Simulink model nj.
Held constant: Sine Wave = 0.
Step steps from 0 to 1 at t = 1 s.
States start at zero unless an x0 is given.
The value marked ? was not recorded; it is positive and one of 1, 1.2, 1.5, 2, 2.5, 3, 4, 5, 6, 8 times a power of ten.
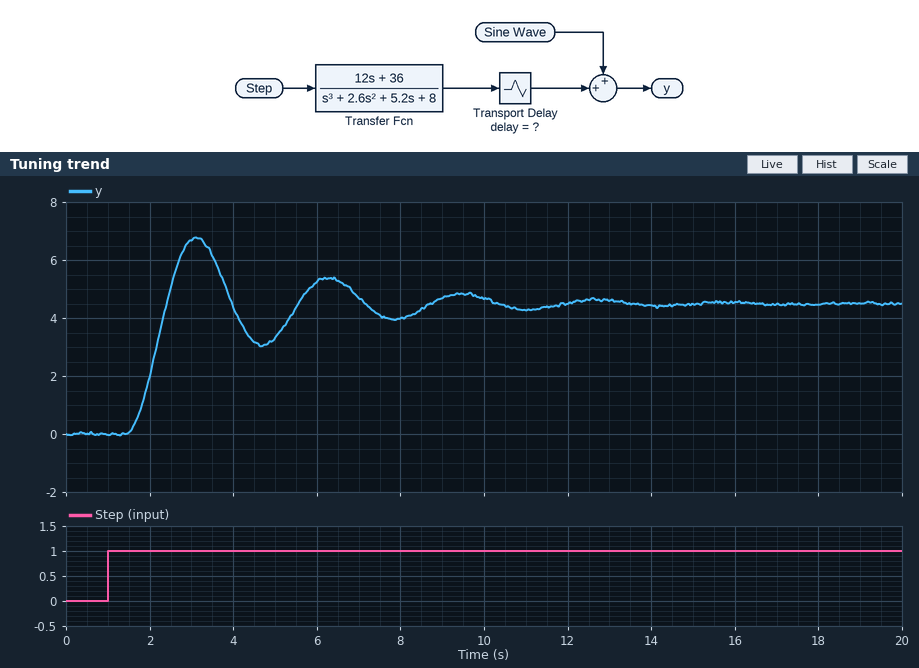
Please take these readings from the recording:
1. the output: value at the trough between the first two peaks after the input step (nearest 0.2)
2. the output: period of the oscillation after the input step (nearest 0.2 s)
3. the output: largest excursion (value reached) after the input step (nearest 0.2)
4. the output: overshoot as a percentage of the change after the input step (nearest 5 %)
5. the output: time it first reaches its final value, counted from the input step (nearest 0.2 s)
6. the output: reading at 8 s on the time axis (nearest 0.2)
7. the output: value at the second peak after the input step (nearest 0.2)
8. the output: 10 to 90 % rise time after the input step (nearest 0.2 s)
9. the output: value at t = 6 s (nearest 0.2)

3.0
3.2 s
6.8
50 %
1.4 s
4.0
5.4
0.6 s
5.2
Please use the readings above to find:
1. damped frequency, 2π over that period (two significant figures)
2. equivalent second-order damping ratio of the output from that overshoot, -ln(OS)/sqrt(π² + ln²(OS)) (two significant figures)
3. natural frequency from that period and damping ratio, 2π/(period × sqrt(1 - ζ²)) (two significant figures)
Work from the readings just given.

2.0 rad/s
0.22
2.0 rad/s
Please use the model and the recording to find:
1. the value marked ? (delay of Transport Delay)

0.4
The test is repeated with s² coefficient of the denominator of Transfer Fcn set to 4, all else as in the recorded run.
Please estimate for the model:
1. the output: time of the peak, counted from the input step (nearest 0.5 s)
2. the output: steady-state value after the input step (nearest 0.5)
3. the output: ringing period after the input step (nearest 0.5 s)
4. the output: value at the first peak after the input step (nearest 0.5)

2.5 s
4.5
4.0 s
6.5
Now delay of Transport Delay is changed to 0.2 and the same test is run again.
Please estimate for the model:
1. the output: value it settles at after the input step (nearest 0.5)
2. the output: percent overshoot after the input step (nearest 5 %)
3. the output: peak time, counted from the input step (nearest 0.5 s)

4.5
50 %
2.0 s
